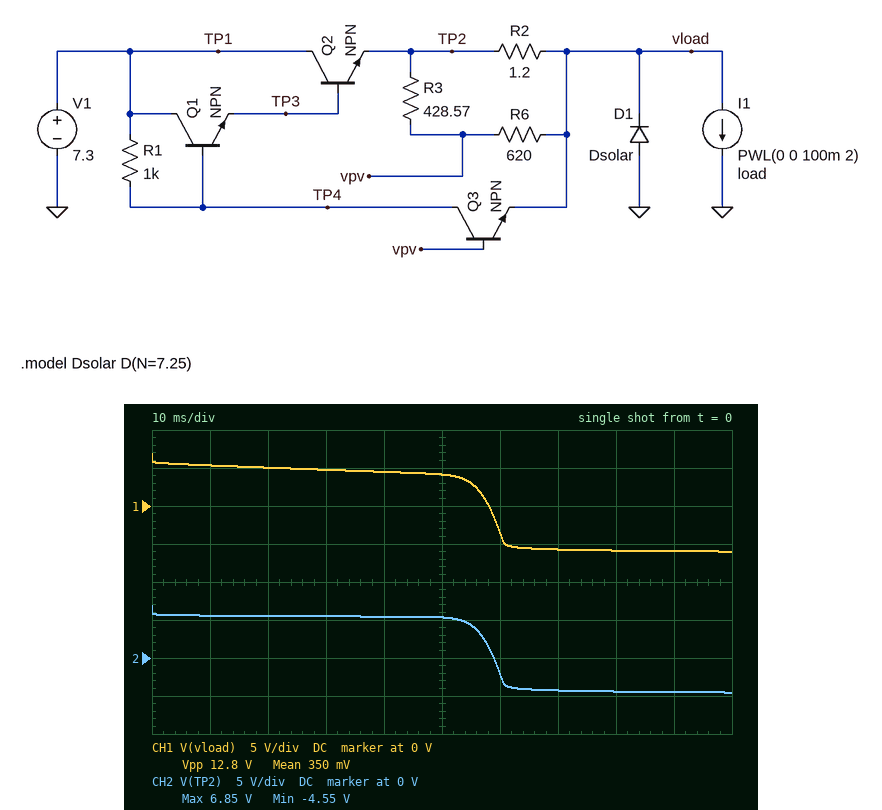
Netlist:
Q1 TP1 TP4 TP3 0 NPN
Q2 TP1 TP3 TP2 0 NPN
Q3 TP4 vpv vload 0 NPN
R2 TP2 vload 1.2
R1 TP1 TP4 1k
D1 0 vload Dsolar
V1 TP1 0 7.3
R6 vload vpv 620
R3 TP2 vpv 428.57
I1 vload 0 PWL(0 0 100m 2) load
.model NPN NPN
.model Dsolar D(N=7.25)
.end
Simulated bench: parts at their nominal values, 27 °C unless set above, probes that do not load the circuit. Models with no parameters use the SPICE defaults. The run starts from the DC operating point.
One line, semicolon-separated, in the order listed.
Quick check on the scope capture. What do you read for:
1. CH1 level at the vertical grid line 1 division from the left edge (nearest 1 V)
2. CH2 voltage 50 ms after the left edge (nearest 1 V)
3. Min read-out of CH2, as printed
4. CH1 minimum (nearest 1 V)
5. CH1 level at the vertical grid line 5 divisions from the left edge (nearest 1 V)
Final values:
5 V; 5 V; -4.55 V; -6 V; 4 V
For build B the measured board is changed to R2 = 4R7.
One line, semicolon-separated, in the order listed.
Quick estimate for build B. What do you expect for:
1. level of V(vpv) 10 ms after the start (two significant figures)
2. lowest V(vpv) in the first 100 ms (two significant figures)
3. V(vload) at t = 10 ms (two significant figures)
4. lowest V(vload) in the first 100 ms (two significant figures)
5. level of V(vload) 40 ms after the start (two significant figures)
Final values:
5.2 V; -5.3 V; 4.6 V; -6.1 V; -5.9 V
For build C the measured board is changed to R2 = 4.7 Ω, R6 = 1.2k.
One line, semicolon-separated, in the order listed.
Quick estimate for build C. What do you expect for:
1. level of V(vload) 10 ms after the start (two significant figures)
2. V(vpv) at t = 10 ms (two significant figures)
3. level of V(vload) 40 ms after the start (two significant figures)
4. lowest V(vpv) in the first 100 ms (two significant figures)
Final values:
4.6 V; 5.3 V; -5.9 V; -5.3 V
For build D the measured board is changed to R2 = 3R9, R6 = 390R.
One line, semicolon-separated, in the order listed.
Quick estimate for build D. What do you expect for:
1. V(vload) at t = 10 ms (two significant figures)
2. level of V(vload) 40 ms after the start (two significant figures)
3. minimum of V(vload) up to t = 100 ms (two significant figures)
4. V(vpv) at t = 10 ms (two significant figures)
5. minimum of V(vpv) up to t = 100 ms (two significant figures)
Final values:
4.8 V; -5.8 V; -6.1 V; 5.2 V; -5.3 V
